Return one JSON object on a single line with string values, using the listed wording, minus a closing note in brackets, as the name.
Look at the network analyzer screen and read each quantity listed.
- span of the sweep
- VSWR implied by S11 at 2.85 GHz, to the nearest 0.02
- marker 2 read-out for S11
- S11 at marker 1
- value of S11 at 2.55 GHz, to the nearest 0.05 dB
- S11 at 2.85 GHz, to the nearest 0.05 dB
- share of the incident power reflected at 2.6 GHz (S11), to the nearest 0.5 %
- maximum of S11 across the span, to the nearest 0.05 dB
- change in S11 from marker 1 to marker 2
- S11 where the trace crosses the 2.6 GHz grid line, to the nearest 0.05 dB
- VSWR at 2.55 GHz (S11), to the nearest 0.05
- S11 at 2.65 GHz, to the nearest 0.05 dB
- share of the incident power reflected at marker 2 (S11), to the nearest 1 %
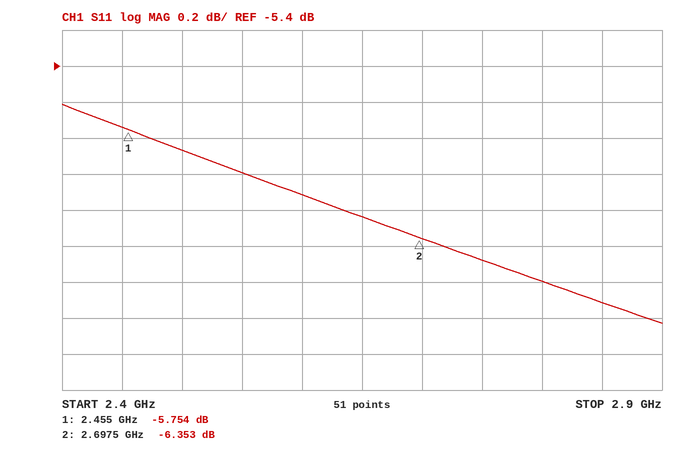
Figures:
{"span of the sweep": "500 MHz", "VSWR implied by S11 at 2.85 GHz, to the nearest 0.02": "2.72", "marker 2 read-out for S11": "-6.353 dB", "S11 at marker 1": "-5.754 dB", "value of S11 at 2.55 GHz, to the nearest 0.05 dB": "-6.00 dB", "S11 at 2.85 GHz, to the nearest 0.05 dB": "-6.70 dB", "share of the incident power reflected at 2.6 GHz (S11), to the nearest 0.5 %": "24.5 %", "maximum of S11 across the span, to the nearest 0.05 dB": "-5.60 dB", "change in S11 from marker 1 to marker 2": "-0.599 dB", "S11 where the trace crosses the 2.6 GHz grid line, to the nearest 0.05 dB": "-6.10 dB", "VSWR at 2.55 GHz (S11), to the nearest 0.05": "3.00", "S11 at 2.65 GHz, to the nearest 0.05 dB": "-6.25 dB", "share of the incident power reflected at marker 2 (S11), to the nearest 1 %": "23 %"}
